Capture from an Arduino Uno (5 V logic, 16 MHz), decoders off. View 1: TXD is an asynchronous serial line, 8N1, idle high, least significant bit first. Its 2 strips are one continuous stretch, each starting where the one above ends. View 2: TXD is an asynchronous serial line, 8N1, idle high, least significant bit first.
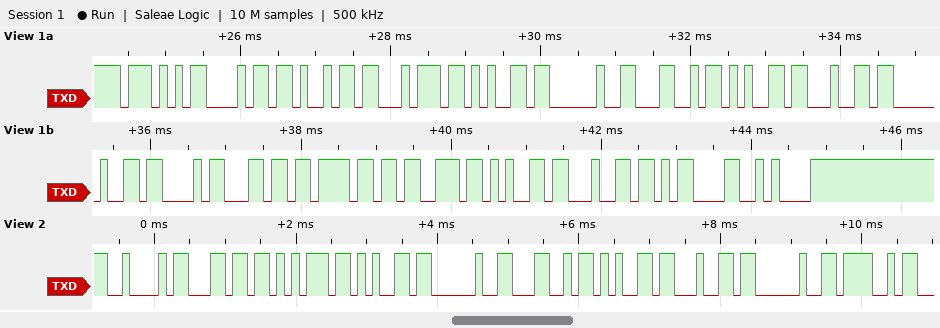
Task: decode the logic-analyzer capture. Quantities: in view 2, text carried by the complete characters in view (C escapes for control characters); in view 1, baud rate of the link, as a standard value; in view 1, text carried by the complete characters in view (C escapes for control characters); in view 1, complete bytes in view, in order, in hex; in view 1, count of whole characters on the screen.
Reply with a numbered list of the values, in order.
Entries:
1. "Blue Led O"
2. 9600 baud
3. "White Led Closed\r\n"
4. 57 68 69 74 65 20 4C 65 64 20 43 6C 6F 73 65 64 0D 0A
5. 18
